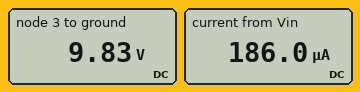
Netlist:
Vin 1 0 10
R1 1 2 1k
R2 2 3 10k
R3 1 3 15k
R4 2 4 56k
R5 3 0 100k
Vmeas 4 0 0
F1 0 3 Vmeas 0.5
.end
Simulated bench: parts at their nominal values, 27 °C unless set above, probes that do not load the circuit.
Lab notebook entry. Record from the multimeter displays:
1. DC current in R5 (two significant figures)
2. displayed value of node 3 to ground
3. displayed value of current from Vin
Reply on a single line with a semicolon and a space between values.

98 µA; 9.83 V; 186.0 µA
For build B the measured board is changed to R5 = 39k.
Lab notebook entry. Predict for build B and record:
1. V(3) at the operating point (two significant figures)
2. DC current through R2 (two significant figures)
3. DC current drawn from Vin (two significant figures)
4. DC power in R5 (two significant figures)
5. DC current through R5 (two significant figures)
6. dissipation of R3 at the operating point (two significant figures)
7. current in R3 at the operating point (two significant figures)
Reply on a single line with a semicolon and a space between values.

9.0 V; 76 µA; 320 µA; 2.1 mW; 230 µA; 68 µW; 67 µA
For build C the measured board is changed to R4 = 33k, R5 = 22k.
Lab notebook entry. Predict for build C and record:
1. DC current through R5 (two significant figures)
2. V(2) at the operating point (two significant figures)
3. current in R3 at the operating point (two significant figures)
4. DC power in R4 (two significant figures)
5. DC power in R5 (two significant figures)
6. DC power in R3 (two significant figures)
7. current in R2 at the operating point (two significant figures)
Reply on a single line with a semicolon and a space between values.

380 µA; 9.6 V; 110 µA; 2.8 mW; 3.2 mW; 180 µW; 120 µA
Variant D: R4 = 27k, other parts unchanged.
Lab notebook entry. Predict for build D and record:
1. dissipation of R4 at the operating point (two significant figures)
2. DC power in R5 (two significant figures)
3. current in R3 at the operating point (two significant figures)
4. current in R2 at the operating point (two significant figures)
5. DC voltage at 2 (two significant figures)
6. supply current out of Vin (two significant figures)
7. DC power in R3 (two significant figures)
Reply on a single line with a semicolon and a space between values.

3.5 mW; 1.1 mW; 19 µA; 58 µA; 9.7 V; 280 µA; 5.2 µW
